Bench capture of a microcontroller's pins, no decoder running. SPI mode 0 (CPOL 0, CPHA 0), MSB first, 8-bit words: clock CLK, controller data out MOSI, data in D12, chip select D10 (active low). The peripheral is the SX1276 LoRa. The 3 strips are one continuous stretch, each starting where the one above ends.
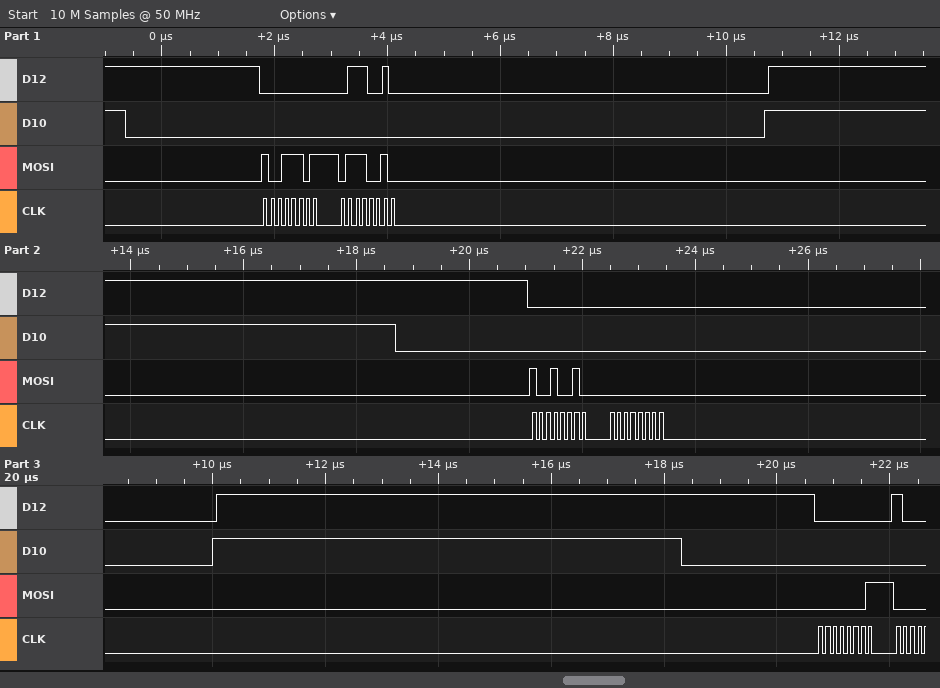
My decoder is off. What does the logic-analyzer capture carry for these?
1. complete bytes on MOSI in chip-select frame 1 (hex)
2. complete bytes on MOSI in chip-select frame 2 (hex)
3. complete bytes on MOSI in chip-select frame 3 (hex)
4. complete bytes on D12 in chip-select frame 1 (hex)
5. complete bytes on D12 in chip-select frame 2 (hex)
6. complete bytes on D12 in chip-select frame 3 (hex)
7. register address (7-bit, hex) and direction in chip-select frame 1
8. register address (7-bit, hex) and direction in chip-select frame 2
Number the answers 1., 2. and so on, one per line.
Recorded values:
1. 0x9D 0x72
2. 0x92 0x00
3. 0x01
4. 0x00 0x72
5. 0x00 0x00
6. 0x00
7. 0x1D write
8. 0x12 write
